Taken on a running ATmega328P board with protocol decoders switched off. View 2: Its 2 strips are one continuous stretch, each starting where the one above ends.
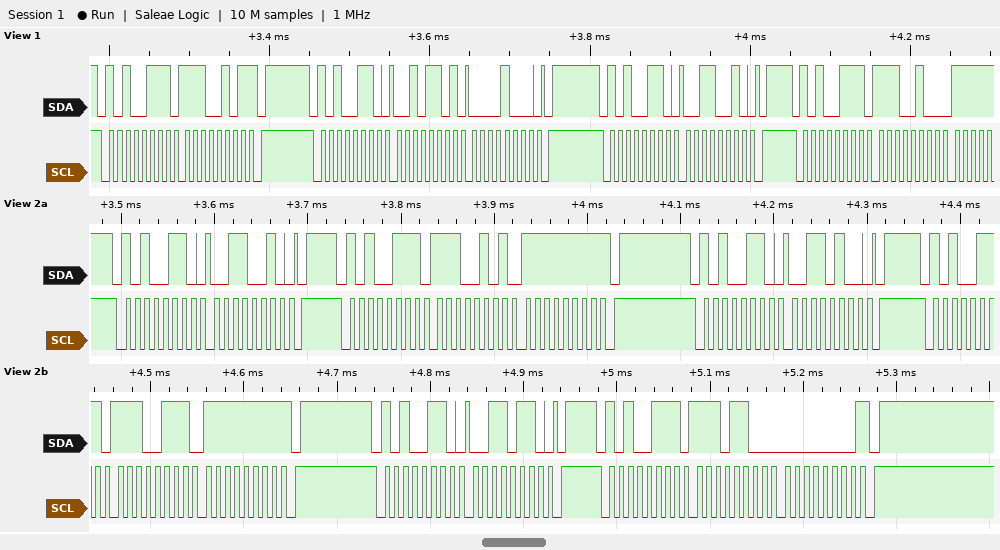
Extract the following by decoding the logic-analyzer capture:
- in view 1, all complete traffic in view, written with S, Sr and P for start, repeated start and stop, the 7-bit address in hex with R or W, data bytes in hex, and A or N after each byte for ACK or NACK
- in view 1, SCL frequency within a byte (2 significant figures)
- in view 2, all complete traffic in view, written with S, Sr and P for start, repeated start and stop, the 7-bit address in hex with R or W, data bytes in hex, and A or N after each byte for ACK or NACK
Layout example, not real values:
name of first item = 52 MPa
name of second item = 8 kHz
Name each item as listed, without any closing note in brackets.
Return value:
in view 1, all complete traffic in view, written with S, Sr and P for start, repeated start and stop, the 7-bit address in hex with R or W, data bytes in hex, and A or N after each byte for ACK or NACK = S 53R A E5 N P S 53W A 2D A 08 A P S 53W A 32 A P S 53R A E4 A
in view 1, SCL frequency within a byte = 100 kHz
in view 2, all complete traffic in view, written with S, Sr and P for start, repeated start and stop, the 7-bit address in hex with R or W, data bytes in hex, and A or N after each byte for ACK or NACK = S 53W A 32 A P S 53R A E5 A FF N P S 53W A 34 A P S 53R A E7 A FF N P S 53W A 36 A P S 53R A EC A 00 N P
